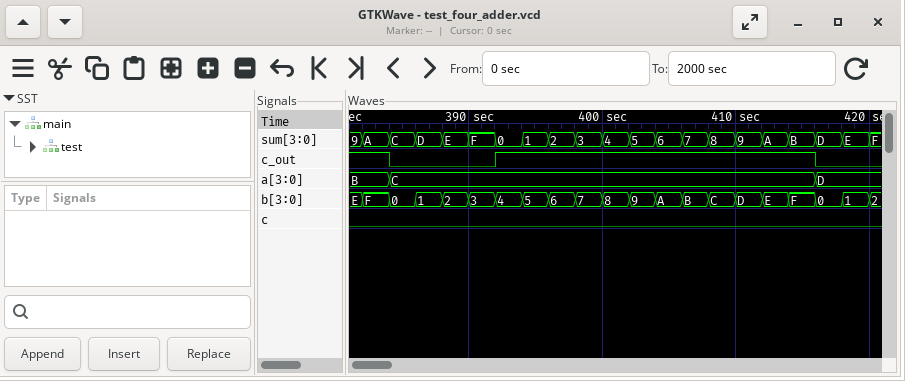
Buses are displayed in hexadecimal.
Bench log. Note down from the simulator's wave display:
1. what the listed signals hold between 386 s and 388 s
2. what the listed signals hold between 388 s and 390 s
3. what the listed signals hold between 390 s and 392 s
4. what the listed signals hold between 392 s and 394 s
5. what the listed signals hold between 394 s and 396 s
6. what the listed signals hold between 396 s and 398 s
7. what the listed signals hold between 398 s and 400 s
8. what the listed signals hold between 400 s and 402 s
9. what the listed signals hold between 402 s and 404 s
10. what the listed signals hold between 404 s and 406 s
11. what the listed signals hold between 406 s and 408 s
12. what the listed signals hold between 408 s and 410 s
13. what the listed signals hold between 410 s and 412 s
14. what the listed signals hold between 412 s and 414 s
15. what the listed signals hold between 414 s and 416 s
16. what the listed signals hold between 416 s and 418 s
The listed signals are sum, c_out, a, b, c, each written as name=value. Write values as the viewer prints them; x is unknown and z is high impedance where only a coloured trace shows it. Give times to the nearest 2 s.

sum=D, c_out=0, a=C, b=1, c=0
sum=E, c_out=0, a=C, b=2, c=0
sum=F, c_out=0, a=C, b=3, c=0
sum=0, c_out=1, a=C, b=4, c=0
sum=1, c_out=1, a=C, b=5, c=0
sum=2, c_out=1, a=C, b=6, c=0
sum=3, c_out=1, a=C, b=7, c=0
sum=4, c_out=1, a=C, b=8, c=0
sum=5, c_out=1, a=C, b=9, c=0
sum=6, c_out=1, a=C, b=A, c=0
sum=7, c_out=1, a=C, b=B, c=0
sum=8, c_out=1, a=C, b=C, c=0
sum=9, c_out=1, a=C, b=D, c=0
sum=A, c_out=1, a=C, b=E, c=0
sum=B, c_out=1, a=C, b=F, c=0
sum=D, c_out=0, a=D, b=0, c=0
